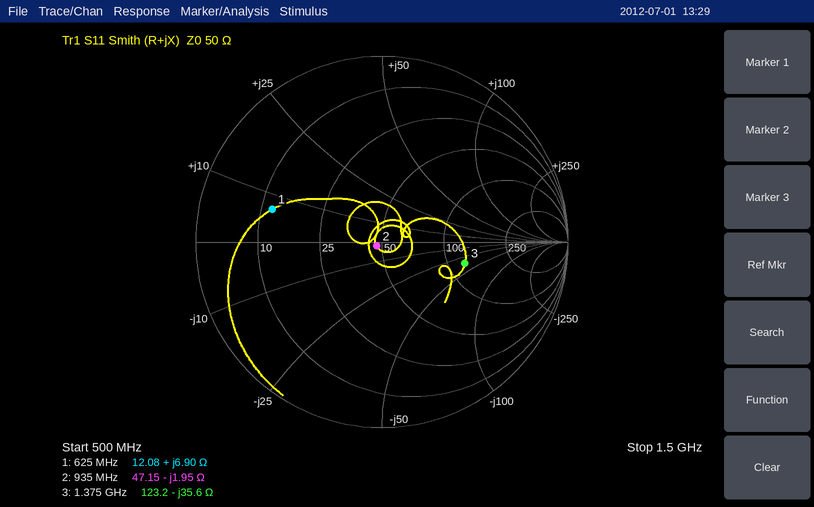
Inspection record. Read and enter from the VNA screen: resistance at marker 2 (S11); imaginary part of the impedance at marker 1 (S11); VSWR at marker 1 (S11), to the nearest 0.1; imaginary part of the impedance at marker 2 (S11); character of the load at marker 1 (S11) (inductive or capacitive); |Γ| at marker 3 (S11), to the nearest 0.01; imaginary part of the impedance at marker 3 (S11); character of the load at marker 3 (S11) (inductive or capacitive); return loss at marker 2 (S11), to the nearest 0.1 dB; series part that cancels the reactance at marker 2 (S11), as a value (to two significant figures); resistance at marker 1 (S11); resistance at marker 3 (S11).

47.15 Ω
+6.90 Ω
4.2
-1.95 Ω
inductive
0.46
-35.6 Ω
capacitive
29.0 dB
330 pH
12.08 Ω
123.2 Ω
